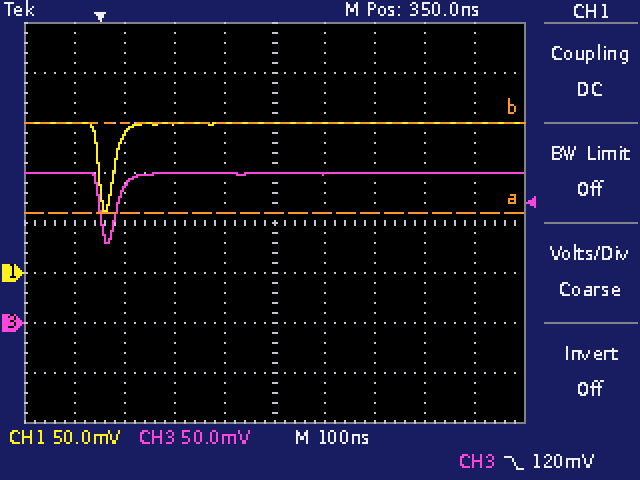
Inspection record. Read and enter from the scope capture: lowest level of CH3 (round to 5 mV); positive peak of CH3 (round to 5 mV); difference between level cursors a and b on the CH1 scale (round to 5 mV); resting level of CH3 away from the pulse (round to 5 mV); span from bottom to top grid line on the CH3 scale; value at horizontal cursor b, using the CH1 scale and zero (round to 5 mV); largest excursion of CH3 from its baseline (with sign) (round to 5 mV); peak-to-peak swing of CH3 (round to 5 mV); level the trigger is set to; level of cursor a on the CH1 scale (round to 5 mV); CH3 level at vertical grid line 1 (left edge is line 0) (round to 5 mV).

80 mV
150 mV
90 mV
150 mV
400 mV
150 mV
-70 mV
70 mV
120 mV
60 mV
150 mV
